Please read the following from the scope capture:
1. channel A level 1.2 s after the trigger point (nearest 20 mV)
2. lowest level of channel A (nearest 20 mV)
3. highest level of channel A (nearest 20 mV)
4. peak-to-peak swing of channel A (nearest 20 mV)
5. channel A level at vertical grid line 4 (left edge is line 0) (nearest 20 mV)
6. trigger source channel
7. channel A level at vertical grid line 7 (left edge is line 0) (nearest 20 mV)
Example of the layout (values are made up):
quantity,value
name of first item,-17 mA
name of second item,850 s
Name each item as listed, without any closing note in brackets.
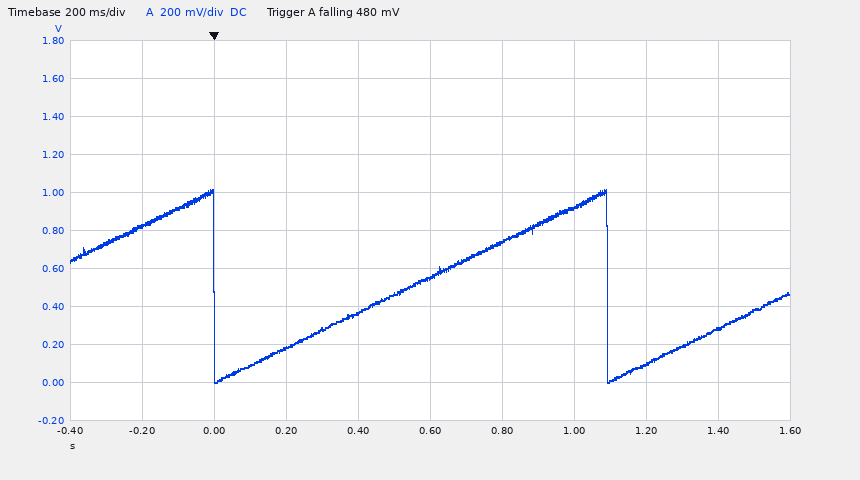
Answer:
quantity,value
channel A level 1.2 s after the trigger point,100 mV
lowest level of channel A,0 mV
highest level of channel A,1.02 V
peak-to-peak swing of channel A,1.02 V
channel A level at vertical grid line 4 (left edge is line 0),360 mV
trigger source channel,channel A
channel A level at vertical grid line 7 (left edge is line 0),920 mV
